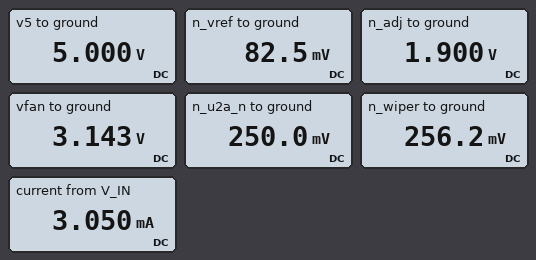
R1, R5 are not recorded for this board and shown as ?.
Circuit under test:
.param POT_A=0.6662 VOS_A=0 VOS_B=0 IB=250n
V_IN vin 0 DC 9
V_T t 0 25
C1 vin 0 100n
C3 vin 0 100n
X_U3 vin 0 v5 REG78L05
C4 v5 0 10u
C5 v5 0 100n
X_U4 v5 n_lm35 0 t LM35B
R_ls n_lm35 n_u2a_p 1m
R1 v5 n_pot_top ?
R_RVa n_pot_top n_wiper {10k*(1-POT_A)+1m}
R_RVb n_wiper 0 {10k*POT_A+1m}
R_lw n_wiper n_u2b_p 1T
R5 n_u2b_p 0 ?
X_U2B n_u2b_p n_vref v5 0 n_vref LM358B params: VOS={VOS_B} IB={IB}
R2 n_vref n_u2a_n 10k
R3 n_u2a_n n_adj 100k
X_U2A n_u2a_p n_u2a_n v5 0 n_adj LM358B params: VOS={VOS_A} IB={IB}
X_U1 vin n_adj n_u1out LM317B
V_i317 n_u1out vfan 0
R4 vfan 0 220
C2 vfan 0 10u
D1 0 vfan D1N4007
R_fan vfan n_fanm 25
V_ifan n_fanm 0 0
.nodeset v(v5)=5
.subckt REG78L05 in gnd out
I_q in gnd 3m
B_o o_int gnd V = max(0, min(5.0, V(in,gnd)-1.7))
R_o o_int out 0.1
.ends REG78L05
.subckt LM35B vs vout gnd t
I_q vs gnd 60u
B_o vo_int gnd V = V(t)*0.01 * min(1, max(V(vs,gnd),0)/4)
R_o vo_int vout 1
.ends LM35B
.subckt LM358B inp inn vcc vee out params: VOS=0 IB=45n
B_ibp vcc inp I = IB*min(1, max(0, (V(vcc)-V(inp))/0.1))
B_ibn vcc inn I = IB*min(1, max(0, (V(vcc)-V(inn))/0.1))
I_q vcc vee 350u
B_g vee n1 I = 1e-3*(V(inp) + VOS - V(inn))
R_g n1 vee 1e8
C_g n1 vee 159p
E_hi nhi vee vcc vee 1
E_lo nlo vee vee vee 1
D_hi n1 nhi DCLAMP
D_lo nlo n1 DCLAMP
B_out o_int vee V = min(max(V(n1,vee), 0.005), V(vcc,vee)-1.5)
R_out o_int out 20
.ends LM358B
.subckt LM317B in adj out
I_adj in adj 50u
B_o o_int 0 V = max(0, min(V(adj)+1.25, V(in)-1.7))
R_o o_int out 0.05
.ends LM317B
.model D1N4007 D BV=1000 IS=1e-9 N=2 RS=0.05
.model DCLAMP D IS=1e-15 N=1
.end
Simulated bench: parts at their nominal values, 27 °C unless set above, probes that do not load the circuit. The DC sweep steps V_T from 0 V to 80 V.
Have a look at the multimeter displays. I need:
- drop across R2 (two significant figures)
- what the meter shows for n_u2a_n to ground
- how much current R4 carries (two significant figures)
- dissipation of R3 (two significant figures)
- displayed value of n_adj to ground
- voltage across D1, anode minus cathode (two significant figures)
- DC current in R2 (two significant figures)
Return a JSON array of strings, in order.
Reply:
["170 mV", "250.0 mV", "14 mA", "27 µW", "1.900 V", "-3.1 V", "17 µA"]
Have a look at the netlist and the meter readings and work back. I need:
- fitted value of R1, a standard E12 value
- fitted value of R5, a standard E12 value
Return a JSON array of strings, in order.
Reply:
["120 kΩ", "330 kΩ"]
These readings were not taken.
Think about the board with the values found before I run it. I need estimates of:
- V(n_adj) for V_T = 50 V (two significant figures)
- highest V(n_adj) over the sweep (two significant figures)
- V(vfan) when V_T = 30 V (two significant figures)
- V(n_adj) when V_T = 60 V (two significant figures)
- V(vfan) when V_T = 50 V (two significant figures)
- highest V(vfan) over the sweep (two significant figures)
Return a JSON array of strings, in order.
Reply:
["3.5 V", "3.5 V", "3.7 V", "3.5 V", "4.7 V", "4.7 V"]
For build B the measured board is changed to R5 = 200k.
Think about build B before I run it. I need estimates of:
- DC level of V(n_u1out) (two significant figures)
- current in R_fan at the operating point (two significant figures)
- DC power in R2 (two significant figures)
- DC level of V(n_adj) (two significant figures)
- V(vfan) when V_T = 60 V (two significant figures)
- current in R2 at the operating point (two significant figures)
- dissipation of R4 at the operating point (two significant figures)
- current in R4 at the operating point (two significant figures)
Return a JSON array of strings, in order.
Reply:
["3.5 V", "140 mA", "4.0 µW", "2.2 V", "4.7 V", "20 µA", "55 mW", "16 mA"]
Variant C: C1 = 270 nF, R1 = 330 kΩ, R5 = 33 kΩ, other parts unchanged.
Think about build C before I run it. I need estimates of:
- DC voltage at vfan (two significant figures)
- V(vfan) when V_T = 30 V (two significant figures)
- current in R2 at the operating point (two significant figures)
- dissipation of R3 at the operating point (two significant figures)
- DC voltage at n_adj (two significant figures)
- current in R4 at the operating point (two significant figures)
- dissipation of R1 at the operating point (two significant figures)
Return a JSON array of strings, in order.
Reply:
["3.9 V", "4.4 V", "24 µA", "57 µW", "2.6 V", "18 mA", "71 µW"]
